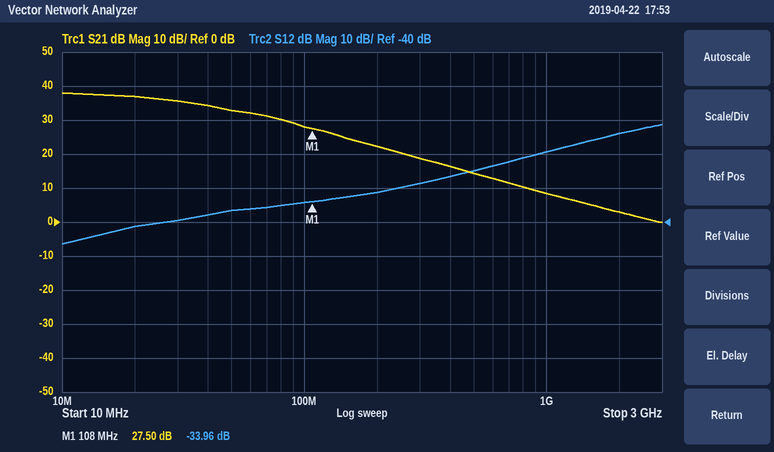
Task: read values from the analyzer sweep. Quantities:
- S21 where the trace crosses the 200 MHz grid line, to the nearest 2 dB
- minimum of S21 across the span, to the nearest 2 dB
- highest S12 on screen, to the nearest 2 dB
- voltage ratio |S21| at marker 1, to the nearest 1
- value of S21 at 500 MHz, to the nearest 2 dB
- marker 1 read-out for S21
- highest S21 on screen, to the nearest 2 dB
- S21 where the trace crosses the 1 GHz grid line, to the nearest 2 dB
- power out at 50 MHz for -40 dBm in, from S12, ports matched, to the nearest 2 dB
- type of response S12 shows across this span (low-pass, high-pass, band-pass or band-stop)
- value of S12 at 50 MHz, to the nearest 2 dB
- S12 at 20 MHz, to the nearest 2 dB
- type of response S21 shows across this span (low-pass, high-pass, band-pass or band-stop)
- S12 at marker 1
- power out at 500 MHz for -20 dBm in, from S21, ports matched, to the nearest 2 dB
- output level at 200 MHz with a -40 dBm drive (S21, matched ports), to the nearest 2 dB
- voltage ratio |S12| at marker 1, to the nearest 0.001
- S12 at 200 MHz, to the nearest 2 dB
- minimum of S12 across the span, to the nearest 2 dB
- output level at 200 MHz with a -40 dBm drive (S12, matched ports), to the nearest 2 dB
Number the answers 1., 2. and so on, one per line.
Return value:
1. 22 dB
2. 0 dB
3. -12 dB
4. 24
5. 14 dB
6. 27.50 dB
7. 38 dB
8. 8 dB
9. -76 dBm
10. high-pass
11. -36 dB
12. -42 dB
13. low-pass
14. -33.96 dB
15. -6 dBm
16. -18 dBm
17. 0.020
18. -32 dB
19. -46 dB
20. -72 dBm
